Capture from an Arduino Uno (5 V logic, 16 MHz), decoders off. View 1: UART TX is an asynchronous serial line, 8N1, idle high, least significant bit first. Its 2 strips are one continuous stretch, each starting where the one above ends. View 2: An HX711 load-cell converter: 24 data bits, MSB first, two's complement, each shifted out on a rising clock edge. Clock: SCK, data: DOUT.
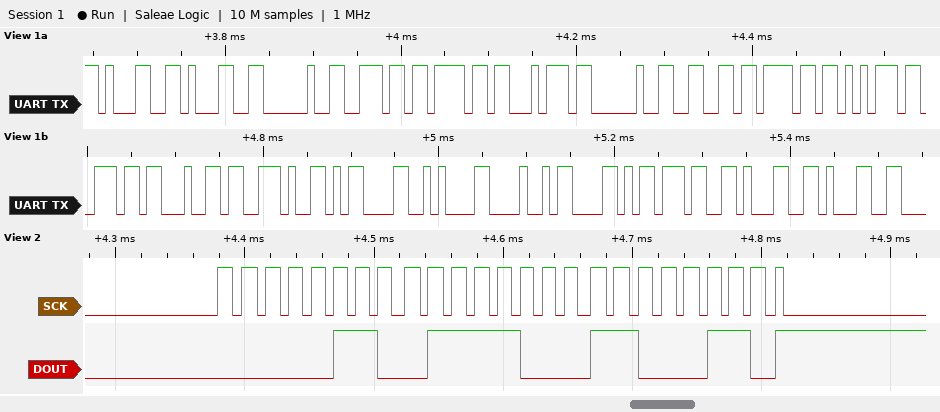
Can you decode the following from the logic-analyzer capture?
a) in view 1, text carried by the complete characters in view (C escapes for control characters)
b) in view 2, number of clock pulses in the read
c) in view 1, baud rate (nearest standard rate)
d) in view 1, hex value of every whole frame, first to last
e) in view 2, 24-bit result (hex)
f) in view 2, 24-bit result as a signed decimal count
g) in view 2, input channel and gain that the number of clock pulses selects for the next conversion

"11 not found.\r\nHX711"
25
115200 baud
0x31 0x31 0x20 0x6E 0x6F 0x74 0x20 0x66 0x6F 0x75 0x6E 0x64 0x2E 0x0D 0x0A 0x48 0x58 0x37 0x31 0x31
0x0678C6
424134
channel A, gain 128
